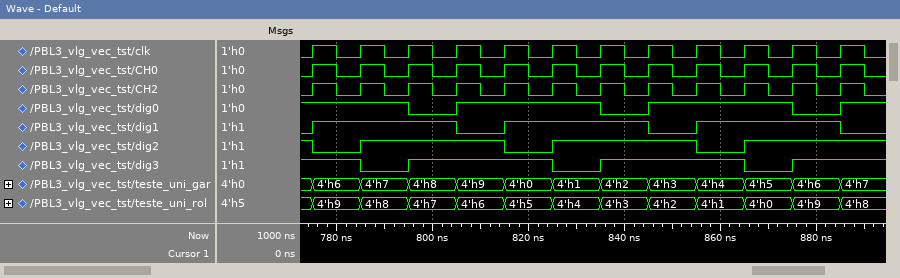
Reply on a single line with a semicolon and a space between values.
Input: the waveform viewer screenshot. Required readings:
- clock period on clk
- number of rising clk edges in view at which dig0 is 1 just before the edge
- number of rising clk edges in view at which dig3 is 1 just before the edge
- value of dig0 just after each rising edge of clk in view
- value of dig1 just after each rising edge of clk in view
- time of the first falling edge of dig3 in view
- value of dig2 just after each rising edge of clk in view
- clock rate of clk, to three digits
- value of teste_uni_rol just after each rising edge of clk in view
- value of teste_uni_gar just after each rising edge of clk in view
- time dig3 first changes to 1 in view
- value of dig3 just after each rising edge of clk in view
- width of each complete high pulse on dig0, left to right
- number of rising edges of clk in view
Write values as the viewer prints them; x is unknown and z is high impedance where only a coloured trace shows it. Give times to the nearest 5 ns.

10 ns; 9; 9; 1 1 0 1 1 1 0 1 1 1 0 1; 1 1 1 0 1 1 1 0 1 1 1 0; 785 ns; 0 1 1 1 0 1 1 1 0 1 1 1; 100 MHz; 4'h9, 4'h8, 4'h7, 4'h6, 4'h5, 4'h4, 4'h3, 4'h2, 4'h1, 4'h0, 4'h9, 4'h8; 4'h6, 4'h7, 4'h8, 4'h9, 4'h0, 4'h1, 4'h2, 4'h3, 4'h4, 4'h5, 4'h6, 4'h7; 795 ns; 1 0 1 1 1 0 1 1 1 0 1 1; 30 ns, 30 ns; 12
